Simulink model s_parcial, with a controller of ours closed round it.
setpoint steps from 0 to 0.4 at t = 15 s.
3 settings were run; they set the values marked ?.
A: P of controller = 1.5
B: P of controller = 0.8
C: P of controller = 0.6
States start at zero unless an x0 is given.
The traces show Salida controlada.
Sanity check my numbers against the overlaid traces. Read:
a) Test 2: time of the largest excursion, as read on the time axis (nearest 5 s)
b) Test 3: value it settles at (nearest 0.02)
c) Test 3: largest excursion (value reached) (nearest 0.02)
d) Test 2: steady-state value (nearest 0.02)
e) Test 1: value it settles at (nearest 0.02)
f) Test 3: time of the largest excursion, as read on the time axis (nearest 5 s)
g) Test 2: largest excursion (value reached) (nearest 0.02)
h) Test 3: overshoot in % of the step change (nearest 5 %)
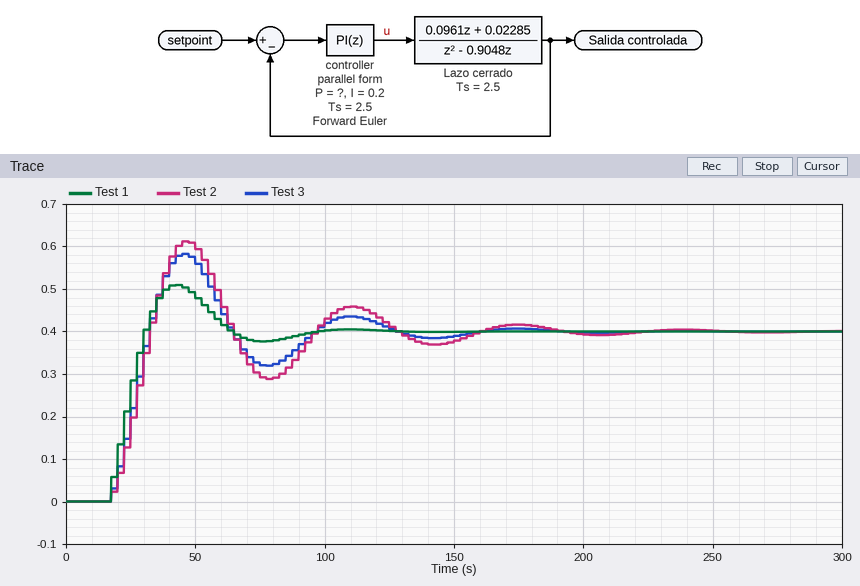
45 s
0.40
0.58
0.40
0.40
45 s
0.62
45 %
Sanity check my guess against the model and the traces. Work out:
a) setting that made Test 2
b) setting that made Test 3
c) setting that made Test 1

C
B
A
